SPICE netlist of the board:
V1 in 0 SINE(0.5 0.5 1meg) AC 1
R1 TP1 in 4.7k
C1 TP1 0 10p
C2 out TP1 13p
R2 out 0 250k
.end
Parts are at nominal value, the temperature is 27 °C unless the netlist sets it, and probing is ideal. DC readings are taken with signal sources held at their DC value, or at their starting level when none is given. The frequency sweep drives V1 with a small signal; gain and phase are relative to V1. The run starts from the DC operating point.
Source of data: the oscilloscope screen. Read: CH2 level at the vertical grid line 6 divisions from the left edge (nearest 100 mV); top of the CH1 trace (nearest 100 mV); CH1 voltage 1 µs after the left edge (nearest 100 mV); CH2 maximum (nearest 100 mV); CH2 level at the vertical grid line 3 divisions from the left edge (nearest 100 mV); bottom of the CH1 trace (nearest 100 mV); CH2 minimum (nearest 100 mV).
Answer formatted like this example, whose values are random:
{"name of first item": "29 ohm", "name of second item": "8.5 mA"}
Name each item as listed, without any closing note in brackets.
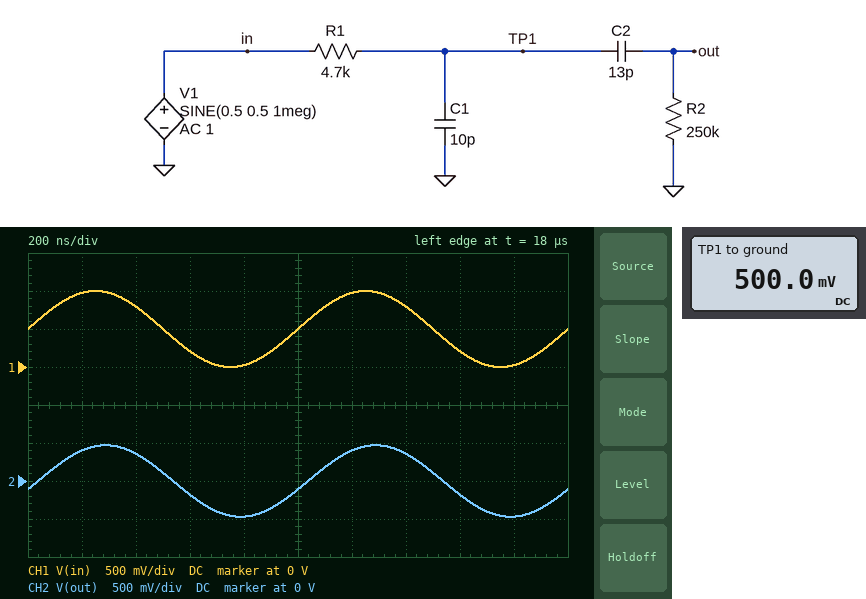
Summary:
{"CH2 level at the vertical grid line 6 divisions from the left edge": "400 mV", "top of the CH1 trace": "1.0 V", "CH1 voltage 1 µs after the left edge": "500 mV", "CH2 maximum": "500 mV", "CH2 level at the vertical grid line 3 divisions from the left edge": "-200 mV", "bottom of the CH1 trace": "0 V", "CH2 minimum": "-500 mV"}
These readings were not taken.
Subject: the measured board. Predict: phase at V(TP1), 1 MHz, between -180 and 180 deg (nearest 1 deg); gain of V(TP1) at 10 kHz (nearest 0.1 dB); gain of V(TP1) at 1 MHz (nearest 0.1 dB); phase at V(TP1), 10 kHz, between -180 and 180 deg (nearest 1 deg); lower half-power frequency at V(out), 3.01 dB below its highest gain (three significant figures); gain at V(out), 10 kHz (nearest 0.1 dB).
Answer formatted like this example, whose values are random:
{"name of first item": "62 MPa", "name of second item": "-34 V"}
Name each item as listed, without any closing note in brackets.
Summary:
{"phase at V(TP1), 1 MHz, between -180 and 180 deg": "-16 deg", "gain of V(TP1) at 10 kHz": "0 dB", "gain of V(TP1) at 1 MHz": "-0.5 dB", "phase at V(TP1), 10 kHz, between -180 and 180 deg": "0 deg", "lower half-power frequency at V(out), 3.01 dB below its highest gain": "46.8 kHz", "gain at V(out), 10 kHz": "-14.0 dB"}
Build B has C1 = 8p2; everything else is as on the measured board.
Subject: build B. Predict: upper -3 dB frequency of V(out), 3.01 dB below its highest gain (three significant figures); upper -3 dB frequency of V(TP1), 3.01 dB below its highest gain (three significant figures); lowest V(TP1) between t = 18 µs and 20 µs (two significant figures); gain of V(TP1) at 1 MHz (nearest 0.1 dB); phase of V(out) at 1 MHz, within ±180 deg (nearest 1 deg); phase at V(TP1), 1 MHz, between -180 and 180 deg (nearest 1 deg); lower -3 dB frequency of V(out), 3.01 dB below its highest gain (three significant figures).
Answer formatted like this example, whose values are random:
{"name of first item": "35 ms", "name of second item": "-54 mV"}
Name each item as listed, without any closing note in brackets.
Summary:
{"upper -3 dB frequency of V(out), 3.01 dB below its highest gain": "4.30 MHz", "upper -3 dB frequency of V(TP1), 3.01 dB below its highest gain": "4.05 MHz", "lowest V(TP1) between t = 18 µs and 20 µs": "23 mV", "gain of V(TP1) at 1 MHz": "-0.4 dB", "phase of V(out) at 1 MHz, within ±180 deg": "-11 deg", "phase at V(TP1), 1 MHz, between -180 and 180 deg": "-13 deg", "lower -3 dB frequency of V(out), 3.01 dB below its highest gain": "47.0 kHz"}
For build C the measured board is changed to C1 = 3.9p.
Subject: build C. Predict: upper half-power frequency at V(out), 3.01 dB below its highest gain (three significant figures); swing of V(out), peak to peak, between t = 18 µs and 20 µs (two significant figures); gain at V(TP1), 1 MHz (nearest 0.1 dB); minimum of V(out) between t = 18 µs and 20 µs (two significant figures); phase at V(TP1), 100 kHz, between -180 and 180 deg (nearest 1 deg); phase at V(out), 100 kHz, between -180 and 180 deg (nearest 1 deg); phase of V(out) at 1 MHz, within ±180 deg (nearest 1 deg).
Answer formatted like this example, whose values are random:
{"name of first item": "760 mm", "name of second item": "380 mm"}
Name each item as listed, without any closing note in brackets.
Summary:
{"upper half-power frequency at V(out), 3.01 dB below its highest gain": "8.94 MHz", "swing of V(out), peak to peak, between t = 18 µs and 20 µs": "970 mV", "gain at V(TP1), 1 MHz": "-0.2 dB", "minimum of V(out) between t = 18 µs and 20 µs": "-490 mV", "phase at V(TP1), 100 kHz, between -180 and 180 deg": "-1 deg", "phase at V(out), 100 kHz, between -180 and 180 deg": "25 deg", "phase of V(out) at 1 MHz, within ±180 deg": "-4 deg"}
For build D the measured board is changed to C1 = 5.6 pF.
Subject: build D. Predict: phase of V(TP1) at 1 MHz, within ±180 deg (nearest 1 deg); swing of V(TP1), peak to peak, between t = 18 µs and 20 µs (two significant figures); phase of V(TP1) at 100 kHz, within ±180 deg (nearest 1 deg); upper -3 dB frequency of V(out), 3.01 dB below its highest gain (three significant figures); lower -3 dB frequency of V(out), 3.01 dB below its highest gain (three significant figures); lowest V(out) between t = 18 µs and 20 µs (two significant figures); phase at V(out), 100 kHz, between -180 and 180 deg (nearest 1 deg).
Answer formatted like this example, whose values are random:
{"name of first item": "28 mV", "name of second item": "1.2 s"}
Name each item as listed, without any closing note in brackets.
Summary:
{"phase of V(TP1) at 1 MHz, within ±180 deg": "-9 deg", "swing of V(TP1), peak to peak, between t = 18 µs and 20 µs": "970 mV", "phase of V(TP1) at 100 kHz, within ±180 deg": "-1 deg", "upper -3 dB frequency of V(out), 3.01 dB below its highest gain": "6.26 MHz", "lower -3 dB frequency of V(out), 3.01 dB below its highest gain": "47.3 kHz", "lowest V(out) between t = 18 µs and 20 µs": "-480 mV", "phase at V(out), 100 kHz, between -180 and 180 deg": "25 deg"}
